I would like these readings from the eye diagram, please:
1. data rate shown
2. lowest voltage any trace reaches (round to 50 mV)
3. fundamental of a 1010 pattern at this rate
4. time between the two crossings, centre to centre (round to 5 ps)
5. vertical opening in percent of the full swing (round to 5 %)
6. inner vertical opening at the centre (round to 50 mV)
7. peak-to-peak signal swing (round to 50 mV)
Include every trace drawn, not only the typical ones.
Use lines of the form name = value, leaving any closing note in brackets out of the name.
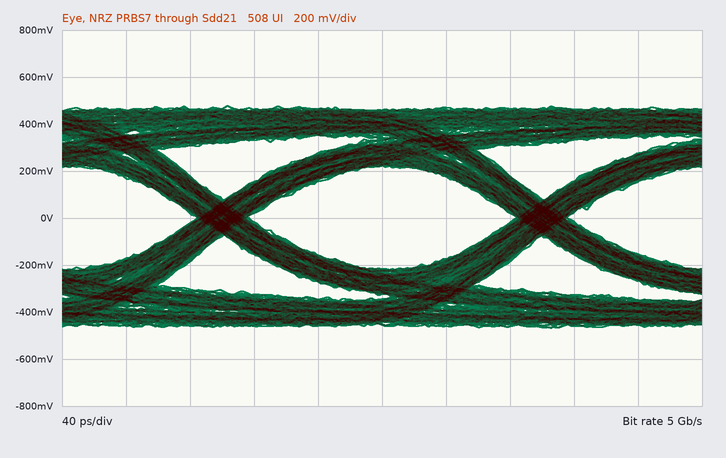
data rate shown = 5 Gb/s
lowest voltage any trace reaches = -450 mV
fundamental of a 1010 pattern at this rate = 2.5 GHz
time between the two crossings, centre to centre = 200 ps
vertical opening in percent of the full swing = 45 %
inner vertical opening at the centre = 450 mV
peak-to-peak signal swing = 950 mV
